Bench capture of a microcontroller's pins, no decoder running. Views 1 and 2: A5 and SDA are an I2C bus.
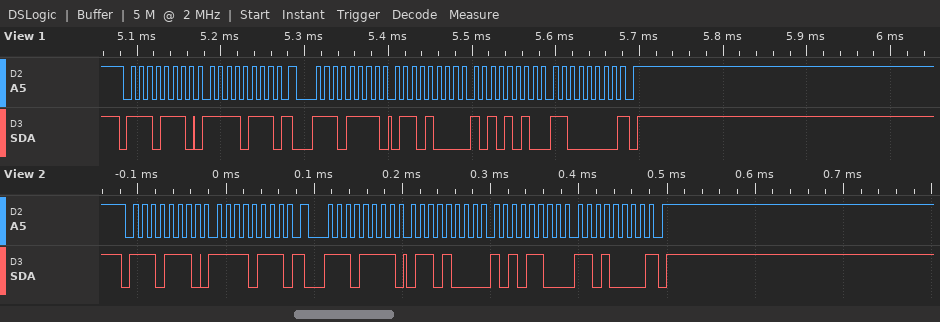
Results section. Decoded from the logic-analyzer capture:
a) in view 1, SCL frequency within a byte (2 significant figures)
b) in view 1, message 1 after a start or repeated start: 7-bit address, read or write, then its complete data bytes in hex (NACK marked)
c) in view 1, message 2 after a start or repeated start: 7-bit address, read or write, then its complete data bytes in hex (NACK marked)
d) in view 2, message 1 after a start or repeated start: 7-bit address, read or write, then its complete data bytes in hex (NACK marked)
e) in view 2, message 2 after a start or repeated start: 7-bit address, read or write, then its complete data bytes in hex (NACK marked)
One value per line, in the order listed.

100 kHz
0x77 write: F7
0x77 read: 68 AA C0 NACK
0x77 write: F7
0x77 read: 68 AC D0 NACK
